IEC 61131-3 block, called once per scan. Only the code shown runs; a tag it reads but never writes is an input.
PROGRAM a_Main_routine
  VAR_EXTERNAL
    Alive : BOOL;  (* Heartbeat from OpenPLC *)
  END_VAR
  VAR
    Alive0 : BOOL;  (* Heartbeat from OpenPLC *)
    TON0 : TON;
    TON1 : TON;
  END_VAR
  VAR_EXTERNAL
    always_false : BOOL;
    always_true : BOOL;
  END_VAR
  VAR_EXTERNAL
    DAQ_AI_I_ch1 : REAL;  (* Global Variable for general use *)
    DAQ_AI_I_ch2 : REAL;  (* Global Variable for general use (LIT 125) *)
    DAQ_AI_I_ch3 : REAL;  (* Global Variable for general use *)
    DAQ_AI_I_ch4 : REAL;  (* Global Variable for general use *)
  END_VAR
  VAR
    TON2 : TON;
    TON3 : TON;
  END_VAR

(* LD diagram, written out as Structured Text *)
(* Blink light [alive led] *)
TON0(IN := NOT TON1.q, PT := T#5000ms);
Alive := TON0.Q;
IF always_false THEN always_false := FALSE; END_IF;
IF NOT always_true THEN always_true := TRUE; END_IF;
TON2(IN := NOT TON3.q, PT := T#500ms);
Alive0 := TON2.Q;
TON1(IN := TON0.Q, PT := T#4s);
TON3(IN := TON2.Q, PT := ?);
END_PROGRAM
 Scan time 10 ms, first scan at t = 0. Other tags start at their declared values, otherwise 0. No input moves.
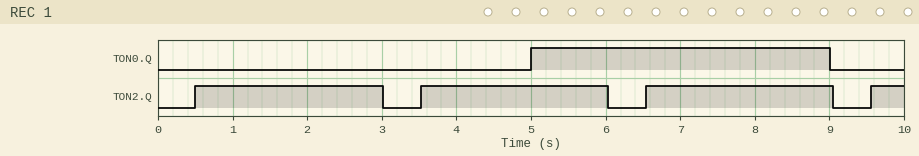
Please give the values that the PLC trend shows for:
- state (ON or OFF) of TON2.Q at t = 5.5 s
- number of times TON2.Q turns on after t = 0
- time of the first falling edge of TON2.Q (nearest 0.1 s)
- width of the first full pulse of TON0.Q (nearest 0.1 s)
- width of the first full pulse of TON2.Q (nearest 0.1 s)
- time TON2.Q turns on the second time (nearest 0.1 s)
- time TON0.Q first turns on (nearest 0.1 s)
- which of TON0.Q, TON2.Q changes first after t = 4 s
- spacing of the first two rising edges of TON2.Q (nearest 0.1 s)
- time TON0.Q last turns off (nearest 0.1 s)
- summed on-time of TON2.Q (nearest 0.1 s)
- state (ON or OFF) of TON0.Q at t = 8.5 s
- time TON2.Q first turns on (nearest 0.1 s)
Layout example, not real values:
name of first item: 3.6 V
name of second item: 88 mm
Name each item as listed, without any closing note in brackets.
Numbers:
state (ON or OFF) of TON2.Q at t = 5.5 s: ON
number of times TON2.Q turns on after t = 0: 4
time of the first falling edge of TON2.Q: 3.0 s
width of the first full pulse of TON0.Q: 4.0 s
width of the first full pulse of TON2.Q: 2.5 s
time TON2.Q turns on the second time: 3.5 s
time TON0.Q first turns on: 5.0 s
which of TON0.Q, TON2.Q changes first after t = 4 s: TON0.Q
spacing of the first two rising edges of TON2.Q: 3.0 s
time TON0.Q last turns off: 9.0 s
summed on-time of TON2.Q: 8.0 s
state (ON or OFF) of TON0.Q at t = 8.5 s: ON
time TON2.Q first turns on: 0.5 s
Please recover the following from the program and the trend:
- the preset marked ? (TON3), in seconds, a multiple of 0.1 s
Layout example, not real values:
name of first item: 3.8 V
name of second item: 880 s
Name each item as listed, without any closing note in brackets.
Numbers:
the preset marked ? (TON3), in seconds, a multiple of 0.1 s: 2.5 s
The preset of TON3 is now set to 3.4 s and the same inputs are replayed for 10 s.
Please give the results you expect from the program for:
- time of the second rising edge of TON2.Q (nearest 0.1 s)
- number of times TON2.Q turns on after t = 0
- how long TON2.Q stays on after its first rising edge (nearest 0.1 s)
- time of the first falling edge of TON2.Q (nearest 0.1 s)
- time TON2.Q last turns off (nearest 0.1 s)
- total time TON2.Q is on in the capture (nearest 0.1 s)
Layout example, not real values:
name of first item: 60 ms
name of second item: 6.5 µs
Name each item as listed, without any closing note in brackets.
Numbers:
time of the second rising edge of TON2.Q: 4.4 s
number of times TON2.Q turns on after t = 0: 3
how long TON2.Q stays on after its first rising edge: 3.4 s
time of the first falling edge of TON2.Q: 3.9 s
time TON2.Q last turns off: 7.8 s
total time TON2.Q is on in the capture: 8.5 s
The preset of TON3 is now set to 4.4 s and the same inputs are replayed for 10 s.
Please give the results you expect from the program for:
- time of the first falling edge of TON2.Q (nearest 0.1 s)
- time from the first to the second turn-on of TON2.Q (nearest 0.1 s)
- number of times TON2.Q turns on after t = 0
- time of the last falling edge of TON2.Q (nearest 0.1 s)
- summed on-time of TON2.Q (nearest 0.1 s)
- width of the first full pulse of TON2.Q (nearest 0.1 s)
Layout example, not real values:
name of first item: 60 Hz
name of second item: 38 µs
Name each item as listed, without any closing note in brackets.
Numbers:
time of the first falling edge of TON2.Q: 4.9 s
time from the first to the second turn-on of TON2.Q: 4.9 s
number of times TON2.Q turns on after t = 0: 2
time of the last falling edge of TON2.Q: 9.8 s
summed on-time of TON2.Q: 8.8 s
width of the first full pulse of TON2.Q: 4.4 s
